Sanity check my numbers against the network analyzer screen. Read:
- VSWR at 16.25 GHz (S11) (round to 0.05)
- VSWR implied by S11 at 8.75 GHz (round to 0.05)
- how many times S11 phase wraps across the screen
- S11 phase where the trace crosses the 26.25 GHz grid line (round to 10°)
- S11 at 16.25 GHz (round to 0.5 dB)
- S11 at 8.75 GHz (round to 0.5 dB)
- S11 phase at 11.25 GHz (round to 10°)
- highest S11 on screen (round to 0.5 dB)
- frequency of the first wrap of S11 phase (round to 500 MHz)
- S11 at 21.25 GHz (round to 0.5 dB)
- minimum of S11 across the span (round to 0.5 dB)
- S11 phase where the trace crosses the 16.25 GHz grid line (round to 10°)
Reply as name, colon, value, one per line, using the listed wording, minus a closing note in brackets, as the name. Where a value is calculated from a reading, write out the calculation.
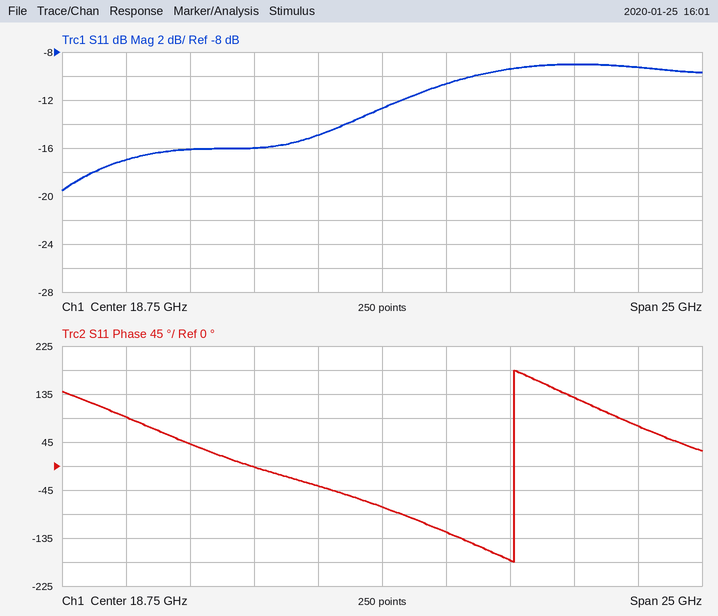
VSWR at 16.25 GHz (S11): |Γ| = 10^(-15/20) = 0.1778; VSWR = (1 + 0.1778)/(1 − 0.1778) ≈ 1.43, so 1.45 to the nearest 0.05
VSWR implied by S11 at 8.75 GHz: |Γ| = 10^(-17/20) = 0.1413; VSWR = (1 + 0.1413)/(1 − 0.1413) ≈ 1.33, so 1.35 to the nearest 0.05
how many times S11 phase wraps across the screen: 1
S11 phase where the trace crosses the 26.25 GHz grid line: 130°
S11 at 16.25 GHz: -15.0 dB
S11 at 8.75 GHz: -17.0 dB
S11 phase at 11.25 GHz: 40°
highest S11 on screen: -9.0 dB
frequency of the first wrap of S11 phase: 24.0 GHz
S11 at 21.25 GHz: -10.5 dB
minimum of S11 across the span: -19.5 dB
S11 phase where the trace crosses the 16.25 GHz grid line: -40°
